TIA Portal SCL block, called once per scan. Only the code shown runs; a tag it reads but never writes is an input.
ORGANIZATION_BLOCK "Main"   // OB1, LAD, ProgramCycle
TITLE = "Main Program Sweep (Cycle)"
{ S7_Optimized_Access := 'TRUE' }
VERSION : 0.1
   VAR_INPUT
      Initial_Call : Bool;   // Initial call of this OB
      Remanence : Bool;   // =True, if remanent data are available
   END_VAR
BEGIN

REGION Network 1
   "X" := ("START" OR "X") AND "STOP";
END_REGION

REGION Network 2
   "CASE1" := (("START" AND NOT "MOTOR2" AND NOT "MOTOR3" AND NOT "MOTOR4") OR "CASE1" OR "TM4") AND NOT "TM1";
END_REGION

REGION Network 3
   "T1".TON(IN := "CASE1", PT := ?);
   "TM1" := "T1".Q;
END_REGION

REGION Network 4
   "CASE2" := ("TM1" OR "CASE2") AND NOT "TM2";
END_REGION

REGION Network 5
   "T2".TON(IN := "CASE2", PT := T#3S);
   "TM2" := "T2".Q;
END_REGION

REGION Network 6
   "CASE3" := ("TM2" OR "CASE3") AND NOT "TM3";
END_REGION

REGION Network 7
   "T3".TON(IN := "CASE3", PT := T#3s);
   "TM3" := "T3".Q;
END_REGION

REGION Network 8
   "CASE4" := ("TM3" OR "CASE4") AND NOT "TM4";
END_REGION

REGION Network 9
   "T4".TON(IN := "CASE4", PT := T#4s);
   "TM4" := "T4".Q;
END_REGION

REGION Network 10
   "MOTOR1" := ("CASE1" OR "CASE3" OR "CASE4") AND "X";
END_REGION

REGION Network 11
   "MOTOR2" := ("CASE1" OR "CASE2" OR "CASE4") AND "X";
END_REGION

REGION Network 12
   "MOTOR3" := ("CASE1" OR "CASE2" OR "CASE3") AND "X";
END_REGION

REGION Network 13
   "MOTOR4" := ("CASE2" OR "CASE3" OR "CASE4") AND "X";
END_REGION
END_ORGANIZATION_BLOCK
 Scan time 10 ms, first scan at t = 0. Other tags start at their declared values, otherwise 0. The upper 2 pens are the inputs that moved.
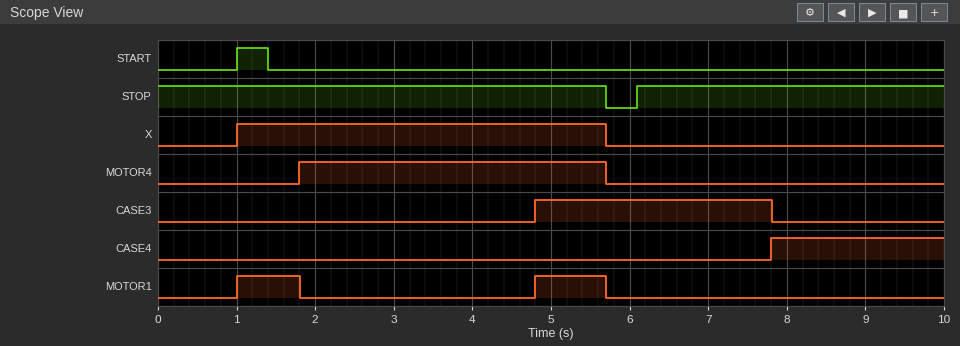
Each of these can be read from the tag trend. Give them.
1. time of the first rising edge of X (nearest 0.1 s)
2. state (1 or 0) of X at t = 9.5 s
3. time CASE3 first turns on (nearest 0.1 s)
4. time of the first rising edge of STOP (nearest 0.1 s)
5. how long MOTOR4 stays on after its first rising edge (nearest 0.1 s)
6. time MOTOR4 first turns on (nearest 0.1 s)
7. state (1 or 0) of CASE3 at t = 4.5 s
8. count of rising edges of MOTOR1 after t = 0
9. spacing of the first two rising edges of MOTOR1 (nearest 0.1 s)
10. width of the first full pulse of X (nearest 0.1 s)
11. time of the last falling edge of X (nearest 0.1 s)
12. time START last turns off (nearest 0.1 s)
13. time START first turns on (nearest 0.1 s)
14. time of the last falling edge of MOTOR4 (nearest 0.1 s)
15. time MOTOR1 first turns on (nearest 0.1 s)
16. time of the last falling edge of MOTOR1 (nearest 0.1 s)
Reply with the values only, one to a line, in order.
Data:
1.0 s
0
4.8 s
6.1 s
3.9 s
1.8 s
0
2
3.8 s
4.7 s
5.7 s
1.4 s
1.0 s
5.7 s
1.0 s
5.7 s
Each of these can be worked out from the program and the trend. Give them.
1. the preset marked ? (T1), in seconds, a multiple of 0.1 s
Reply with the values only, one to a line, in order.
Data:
0.8 s
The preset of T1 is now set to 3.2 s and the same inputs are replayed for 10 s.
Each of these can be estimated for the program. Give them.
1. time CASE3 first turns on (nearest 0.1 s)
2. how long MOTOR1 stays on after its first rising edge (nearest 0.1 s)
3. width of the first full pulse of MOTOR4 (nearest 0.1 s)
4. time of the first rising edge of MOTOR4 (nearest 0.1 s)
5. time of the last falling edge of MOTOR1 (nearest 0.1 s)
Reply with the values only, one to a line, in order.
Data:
7.2 s
3.2 s
1.5 s
4.2 s
4.2 s
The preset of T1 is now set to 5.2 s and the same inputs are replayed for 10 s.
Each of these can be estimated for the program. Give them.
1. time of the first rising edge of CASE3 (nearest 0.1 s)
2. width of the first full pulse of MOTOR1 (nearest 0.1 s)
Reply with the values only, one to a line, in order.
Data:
9.2 s
4.7 s
